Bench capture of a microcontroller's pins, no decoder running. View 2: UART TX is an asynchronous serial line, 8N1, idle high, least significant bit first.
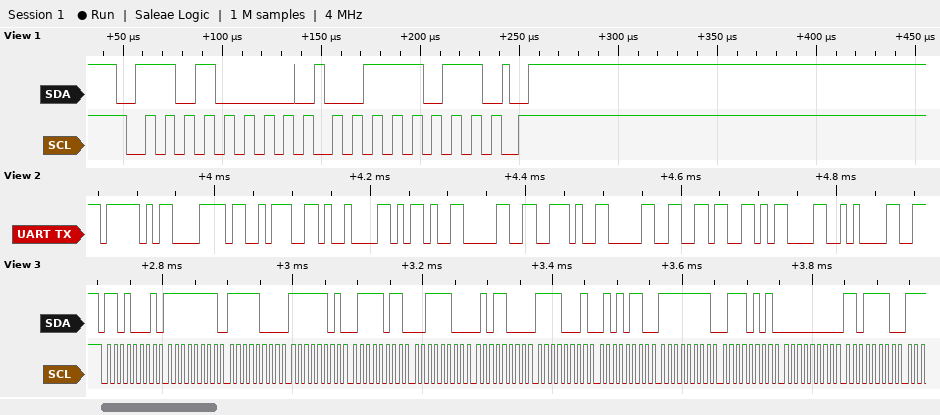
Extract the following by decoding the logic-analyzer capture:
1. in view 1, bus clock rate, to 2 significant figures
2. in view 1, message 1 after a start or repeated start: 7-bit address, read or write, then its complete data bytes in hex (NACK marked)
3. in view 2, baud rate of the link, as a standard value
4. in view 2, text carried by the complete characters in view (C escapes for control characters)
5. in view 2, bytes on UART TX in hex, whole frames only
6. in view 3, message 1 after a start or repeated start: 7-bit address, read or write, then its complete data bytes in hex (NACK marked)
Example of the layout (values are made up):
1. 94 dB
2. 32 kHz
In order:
1. 100 kHz
2. 0x68 write: 3B
3. 115200 baud
4. "_x:\t-0.06\r\n"
5. 5F 78 3A 09 2D 30 2E 30 36 0D 0A
6. 0x68 read: FF F8 FD 7B 3C 58 F1 56 FF 75 00 DE
